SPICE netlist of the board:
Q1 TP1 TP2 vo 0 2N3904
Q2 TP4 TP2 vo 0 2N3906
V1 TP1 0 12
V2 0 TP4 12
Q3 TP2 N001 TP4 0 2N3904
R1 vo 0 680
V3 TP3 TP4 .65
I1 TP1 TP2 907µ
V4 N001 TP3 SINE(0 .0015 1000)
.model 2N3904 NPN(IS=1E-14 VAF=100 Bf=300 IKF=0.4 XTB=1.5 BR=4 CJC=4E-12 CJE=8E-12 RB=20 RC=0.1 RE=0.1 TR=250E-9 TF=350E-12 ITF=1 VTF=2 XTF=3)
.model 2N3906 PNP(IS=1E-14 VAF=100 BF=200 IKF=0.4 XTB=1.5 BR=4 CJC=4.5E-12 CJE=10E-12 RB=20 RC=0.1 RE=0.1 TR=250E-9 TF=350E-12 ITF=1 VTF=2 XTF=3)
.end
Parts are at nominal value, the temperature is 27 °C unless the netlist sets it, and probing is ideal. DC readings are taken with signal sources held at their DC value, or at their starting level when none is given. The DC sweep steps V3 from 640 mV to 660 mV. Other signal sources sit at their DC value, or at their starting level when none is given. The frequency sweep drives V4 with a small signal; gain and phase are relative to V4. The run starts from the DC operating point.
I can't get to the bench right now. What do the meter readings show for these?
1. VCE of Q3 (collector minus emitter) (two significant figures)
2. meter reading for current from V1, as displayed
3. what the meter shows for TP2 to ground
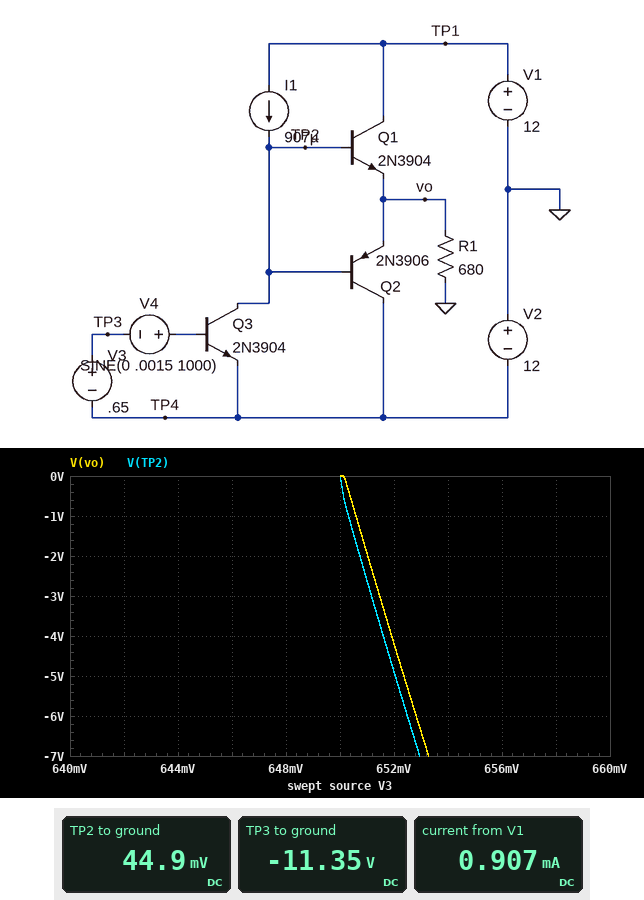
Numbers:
12 V
0.907 mA
44.9 mV
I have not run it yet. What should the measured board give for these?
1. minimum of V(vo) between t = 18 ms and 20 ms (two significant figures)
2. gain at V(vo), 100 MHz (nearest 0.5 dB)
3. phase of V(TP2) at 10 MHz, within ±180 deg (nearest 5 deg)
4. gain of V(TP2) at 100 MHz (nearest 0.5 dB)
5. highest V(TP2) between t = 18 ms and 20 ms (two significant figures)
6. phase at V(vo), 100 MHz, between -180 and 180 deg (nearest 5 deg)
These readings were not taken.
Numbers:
-3.1 V
17.5 dB
115 deg
18.0 dB
4.4 V
100 deg
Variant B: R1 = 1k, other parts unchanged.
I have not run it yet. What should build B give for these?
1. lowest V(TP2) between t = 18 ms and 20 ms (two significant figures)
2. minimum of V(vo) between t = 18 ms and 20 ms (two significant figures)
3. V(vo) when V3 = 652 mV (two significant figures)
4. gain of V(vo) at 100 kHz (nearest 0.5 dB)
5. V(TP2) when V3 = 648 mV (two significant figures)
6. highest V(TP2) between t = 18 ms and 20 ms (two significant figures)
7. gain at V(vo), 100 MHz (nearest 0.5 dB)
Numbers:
-4.3 V
-3.6 V
-4.9 V
27.0 dB
6.5 V
4.9 V
18.5 dB
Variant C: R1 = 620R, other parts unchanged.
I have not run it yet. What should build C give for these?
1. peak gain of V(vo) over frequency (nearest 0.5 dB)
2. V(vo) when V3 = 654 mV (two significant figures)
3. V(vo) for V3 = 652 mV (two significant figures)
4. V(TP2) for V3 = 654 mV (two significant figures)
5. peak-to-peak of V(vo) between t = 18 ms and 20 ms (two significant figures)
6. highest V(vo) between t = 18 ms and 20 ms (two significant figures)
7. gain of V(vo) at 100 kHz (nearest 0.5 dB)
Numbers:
24.0 dB
-8.2 V
-4.0 V
-8.9 V
6.5 V
3.6 V
23.0 dB
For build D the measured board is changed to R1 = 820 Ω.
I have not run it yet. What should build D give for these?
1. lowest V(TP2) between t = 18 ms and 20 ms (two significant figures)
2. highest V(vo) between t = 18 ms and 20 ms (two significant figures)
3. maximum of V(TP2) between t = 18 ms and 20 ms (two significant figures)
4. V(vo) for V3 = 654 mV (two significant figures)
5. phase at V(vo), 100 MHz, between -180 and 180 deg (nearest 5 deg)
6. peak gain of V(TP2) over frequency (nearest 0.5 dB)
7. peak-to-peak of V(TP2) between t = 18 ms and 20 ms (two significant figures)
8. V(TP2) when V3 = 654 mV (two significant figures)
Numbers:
-4.0 V
4.0 V
4.7 V
-9.2 V
95 deg
72.5 dB
8.7 V
-9.9 V
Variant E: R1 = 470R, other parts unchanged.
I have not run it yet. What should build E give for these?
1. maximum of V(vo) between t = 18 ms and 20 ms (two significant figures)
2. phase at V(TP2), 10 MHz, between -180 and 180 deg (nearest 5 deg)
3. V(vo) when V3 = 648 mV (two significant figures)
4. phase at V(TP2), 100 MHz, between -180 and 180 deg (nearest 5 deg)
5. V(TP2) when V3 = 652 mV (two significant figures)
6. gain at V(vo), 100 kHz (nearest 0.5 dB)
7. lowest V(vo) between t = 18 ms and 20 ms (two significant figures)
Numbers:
3.2 V
110 deg
4.3 V
100 deg
-4.2 V
20.5 dB
-2.6 V
